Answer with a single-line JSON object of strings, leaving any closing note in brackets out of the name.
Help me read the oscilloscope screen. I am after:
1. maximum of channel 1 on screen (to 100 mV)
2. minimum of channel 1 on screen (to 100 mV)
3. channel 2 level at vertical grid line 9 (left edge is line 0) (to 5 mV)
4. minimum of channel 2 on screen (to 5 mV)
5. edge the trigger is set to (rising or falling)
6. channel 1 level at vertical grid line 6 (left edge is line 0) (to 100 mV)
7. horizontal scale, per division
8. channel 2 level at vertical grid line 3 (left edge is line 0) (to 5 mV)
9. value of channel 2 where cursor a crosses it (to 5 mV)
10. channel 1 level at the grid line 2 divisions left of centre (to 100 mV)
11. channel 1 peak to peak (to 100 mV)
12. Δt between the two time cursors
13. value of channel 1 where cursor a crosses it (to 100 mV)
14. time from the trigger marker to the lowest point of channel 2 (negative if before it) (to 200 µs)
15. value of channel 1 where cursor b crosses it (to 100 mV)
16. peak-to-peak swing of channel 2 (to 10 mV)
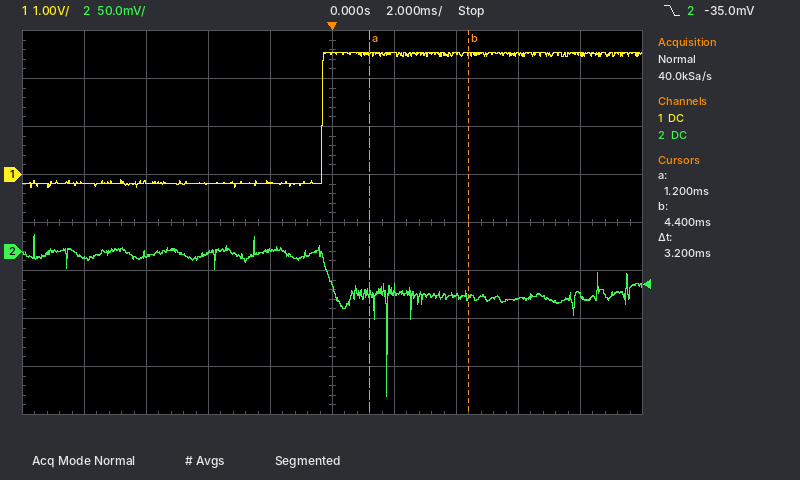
{"maximum of channel 1 on screen": "2.5 V", "minimum of channel 1 on screen": "-300 mV", "channel 2 level at vertical grid line 9 (left edge is line 0)": "-45 mV", "minimum of channel 2 on screen": "-150 mV", "edge the trigger is set to": "falling", "channel 1 level at vertical grid line 6 (left edge is line 0)": "2.5 V", "horizontal scale, per division": "2 ms", "channel 2 level at vertical grid line 3 (left edge is line 0)": "0 mV", "value of channel 2 where cursor a crosses it": "-45 mV", "channel 1 level at the grid line 2 divisions left of centre": "-200 mV", "channel 1 peak to peak": "2.8 V", "Δt between the two time cursors": "3.2 ms", "value of channel 1 where cursor a crosses it": "2.5 V", "time from the trigger marker to the lowest point of channel 2 (negative if before it)": "+1.8 ms", "value of channel 1 where cursor b crosses it": "2.5 V", "peak-to-peak swing of channel 2": "170 mV"}
